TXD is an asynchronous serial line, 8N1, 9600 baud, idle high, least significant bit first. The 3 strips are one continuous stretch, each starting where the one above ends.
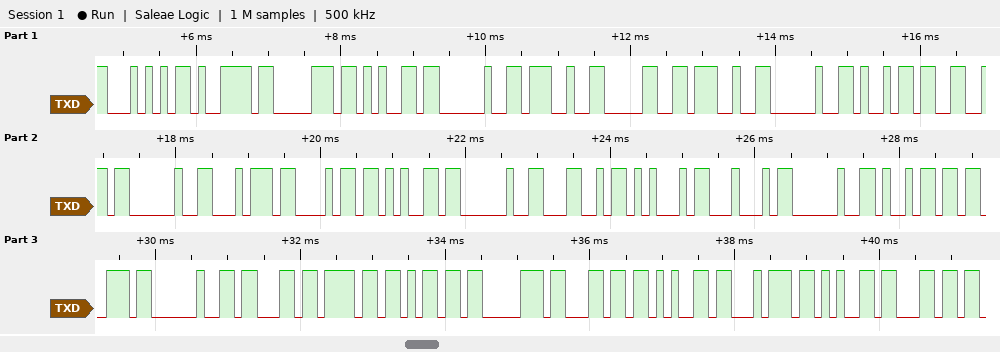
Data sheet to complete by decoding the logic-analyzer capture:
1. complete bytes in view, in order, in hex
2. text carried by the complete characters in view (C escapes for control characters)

54 79 70 65 20 27 30 27 20 69 66 20 74 68 65 20 4C 45 44 20 69 73 20 63 6F 6D 70 6C 65 74 65 6C
"Type '0' if the LED is completel"
